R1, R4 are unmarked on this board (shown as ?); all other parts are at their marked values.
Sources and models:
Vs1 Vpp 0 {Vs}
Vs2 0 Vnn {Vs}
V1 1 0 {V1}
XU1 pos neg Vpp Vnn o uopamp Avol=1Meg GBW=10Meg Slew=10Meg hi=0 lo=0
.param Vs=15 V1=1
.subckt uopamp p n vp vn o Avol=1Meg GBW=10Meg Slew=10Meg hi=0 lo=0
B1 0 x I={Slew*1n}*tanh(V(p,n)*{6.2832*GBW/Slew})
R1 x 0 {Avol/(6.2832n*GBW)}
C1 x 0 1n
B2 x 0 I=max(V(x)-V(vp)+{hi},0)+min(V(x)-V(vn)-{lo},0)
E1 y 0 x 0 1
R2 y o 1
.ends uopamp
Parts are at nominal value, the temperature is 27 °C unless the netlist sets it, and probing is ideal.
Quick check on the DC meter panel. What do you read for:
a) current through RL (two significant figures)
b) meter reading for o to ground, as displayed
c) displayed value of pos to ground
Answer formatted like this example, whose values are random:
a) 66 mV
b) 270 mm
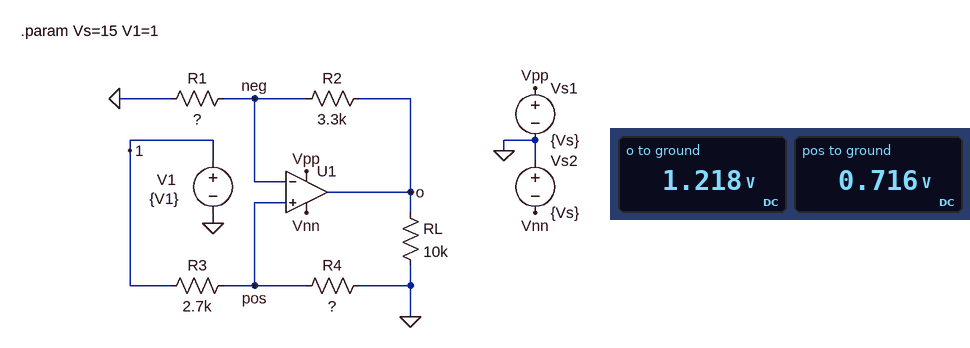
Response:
a) 120 µA
b) 1.218 V
c) 0.716 V
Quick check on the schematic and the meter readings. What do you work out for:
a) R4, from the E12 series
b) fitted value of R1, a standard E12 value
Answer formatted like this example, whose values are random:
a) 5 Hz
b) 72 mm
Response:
a) 6.8 kΩ
b) 4.7 kΩ
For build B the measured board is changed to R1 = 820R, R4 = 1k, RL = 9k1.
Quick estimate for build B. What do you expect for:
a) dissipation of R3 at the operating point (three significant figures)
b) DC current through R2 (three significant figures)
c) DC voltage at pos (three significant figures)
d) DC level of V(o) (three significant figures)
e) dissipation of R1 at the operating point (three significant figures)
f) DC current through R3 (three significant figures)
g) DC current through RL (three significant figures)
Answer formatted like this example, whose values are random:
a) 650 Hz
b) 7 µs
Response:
a) 197 µW
b) 330 µA
c) 270 mV
d) 1.36 V
e) 89.1 µW
f) 270 µA
g) 149 µA
